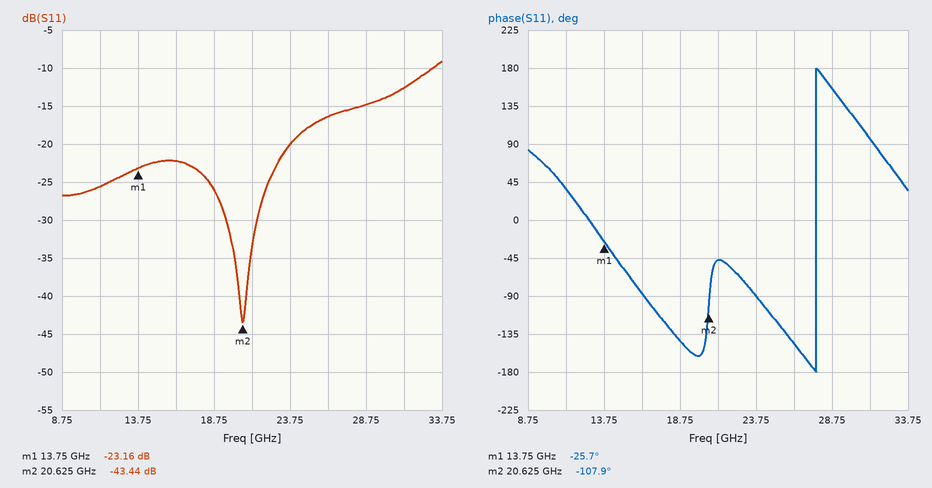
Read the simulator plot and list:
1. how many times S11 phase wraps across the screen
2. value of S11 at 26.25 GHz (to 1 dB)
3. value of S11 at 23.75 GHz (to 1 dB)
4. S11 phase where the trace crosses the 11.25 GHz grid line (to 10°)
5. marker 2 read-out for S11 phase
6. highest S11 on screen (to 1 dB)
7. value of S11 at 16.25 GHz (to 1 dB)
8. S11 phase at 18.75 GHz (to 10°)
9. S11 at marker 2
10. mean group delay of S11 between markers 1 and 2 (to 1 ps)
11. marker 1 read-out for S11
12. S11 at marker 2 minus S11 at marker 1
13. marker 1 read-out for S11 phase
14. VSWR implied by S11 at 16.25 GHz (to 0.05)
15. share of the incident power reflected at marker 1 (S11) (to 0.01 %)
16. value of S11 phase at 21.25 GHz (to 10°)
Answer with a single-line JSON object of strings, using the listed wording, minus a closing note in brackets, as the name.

{"how many times S11 phase wraps across the screen": "1", "value of S11 at 26.25 GHz": "-16 dB", "value of S11 at 23.75 GHz": "-20 dB", "S11 phase where the trace crosses the 11.25 GHz grid line": "40°", "marker 2 read-out for S11 phase": "-107.9°", "highest S11 on screen": "-9 dB", "value of S11 at 16.25 GHz": "-22 dB", "S11 phase at 18.75 GHz": "-140°", "S11 at marker 2": "-43.44 dB", "mean group delay of S11 between markers 1 and 2": "33 ps", "marker 1 read-out for S11": "-23.16 dB", "S11 at marker 2 minus S11 at marker 1": "-20.28 dB", "marker 1 read-out for S11 phase": "-25.7°", "VSWR implied by S11 at 16.25 GHz": "1.15", "share of the incident power reflected at marker 1 (S11)": "0.48 %", "value of S11 phase at 21.25 GHz": "-50°"}
